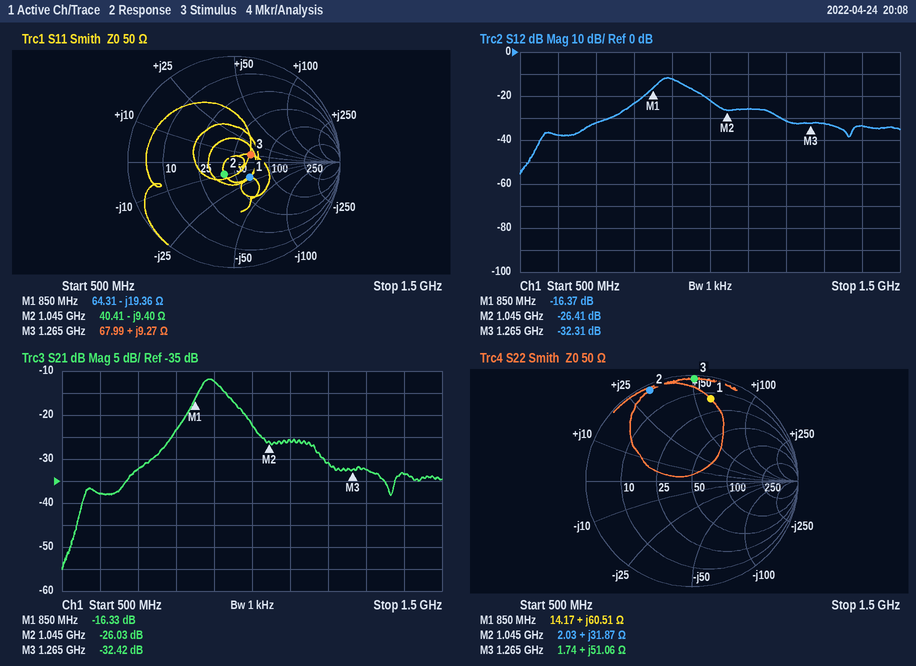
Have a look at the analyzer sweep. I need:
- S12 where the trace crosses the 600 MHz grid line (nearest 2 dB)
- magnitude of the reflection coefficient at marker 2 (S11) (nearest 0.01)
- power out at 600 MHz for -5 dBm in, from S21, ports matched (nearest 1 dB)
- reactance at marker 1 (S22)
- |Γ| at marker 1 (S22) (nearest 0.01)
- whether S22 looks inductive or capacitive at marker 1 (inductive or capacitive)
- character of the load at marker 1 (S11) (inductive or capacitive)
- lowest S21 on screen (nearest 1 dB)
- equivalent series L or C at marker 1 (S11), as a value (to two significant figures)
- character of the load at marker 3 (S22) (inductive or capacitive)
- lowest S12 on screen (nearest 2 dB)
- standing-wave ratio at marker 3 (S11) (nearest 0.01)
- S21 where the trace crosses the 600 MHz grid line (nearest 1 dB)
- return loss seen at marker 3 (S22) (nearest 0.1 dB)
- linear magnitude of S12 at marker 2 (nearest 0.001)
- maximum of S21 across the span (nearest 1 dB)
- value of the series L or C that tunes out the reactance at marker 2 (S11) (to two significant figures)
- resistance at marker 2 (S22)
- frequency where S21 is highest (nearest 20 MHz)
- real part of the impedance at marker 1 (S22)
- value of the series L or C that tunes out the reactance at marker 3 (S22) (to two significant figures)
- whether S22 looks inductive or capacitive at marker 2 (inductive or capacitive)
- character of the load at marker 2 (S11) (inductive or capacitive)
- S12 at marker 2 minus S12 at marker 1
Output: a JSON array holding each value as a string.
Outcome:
["-38 dB", "0.15", "-43 dBm", "+60.51 Ω", "0.80", "inductive", "capacitive", "-55 dB", "9.7 pF", "inductive", "-56 dB", "1.41", "-38 dB", "0.3 dB", "0.048", "-12 dB", "1.4 nH", "2.03 Ω", "880 MHz", "14.17 Ω", "2.5 pF", "inductive", "capacitive", "-10.04 dB"]
